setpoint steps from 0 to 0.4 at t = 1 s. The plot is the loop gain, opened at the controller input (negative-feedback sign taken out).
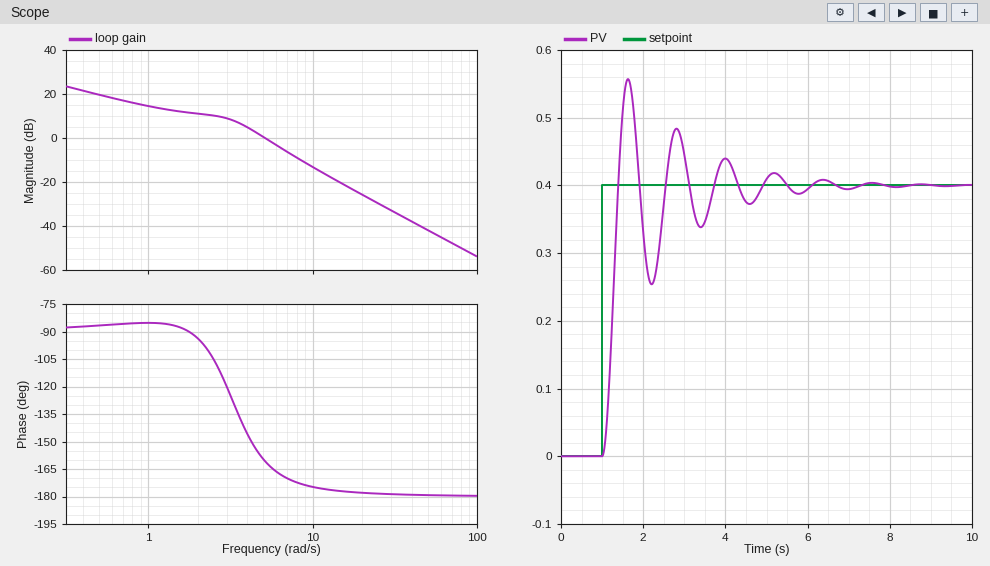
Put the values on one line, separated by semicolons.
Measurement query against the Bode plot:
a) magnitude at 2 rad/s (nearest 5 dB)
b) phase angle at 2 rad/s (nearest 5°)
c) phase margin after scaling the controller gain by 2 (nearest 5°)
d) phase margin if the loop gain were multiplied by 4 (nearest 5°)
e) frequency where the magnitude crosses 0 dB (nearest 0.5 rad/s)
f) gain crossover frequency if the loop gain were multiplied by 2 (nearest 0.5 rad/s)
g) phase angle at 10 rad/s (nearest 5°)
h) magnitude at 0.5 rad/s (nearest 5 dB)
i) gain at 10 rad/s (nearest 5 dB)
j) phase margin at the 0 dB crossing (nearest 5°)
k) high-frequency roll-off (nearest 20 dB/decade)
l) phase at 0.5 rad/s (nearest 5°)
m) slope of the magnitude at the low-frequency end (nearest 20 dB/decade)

10 dB; -95°; 10°; 5°; 5.0 rad/s; 7.0 rad/s; -175°; 20 dB; -15 dB; 20°; -40 dB/decade; -85°; -20 dB/decade
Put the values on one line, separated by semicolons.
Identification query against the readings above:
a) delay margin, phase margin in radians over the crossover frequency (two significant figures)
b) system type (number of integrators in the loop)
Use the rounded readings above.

0.070 s; 1
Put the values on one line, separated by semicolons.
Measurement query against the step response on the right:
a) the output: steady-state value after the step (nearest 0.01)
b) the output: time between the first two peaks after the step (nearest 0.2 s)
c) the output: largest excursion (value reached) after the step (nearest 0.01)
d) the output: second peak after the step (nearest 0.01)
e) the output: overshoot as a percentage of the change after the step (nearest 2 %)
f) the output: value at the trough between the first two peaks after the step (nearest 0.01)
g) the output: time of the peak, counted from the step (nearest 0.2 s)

0.40; 1.2 s; 0.56; 0.48; 40 %; 0.25; 0.6 s
